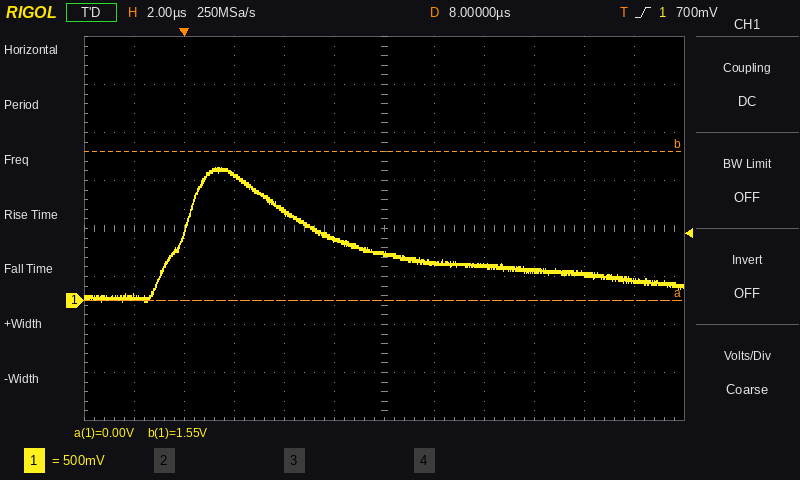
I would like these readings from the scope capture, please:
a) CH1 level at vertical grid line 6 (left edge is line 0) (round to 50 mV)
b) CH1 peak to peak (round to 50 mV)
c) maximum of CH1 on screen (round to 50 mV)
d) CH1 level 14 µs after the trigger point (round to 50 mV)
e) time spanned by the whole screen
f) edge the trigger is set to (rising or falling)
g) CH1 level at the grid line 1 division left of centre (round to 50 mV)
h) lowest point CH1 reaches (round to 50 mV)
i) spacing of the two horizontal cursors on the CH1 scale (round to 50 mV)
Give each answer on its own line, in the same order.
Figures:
500 mV
1.40 V
1.40 V
300 mV
24 µs
rising
650 mV
0 mV
1.55 V
